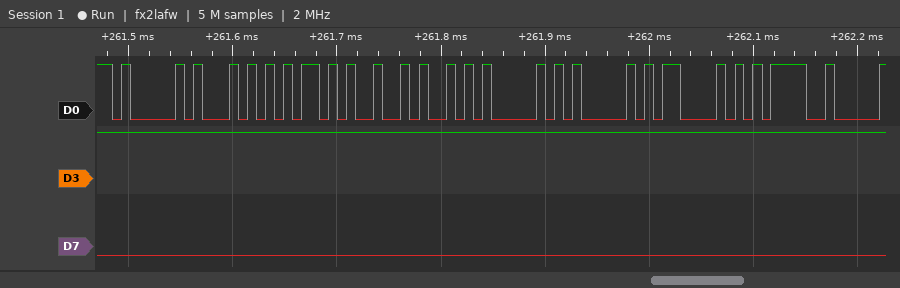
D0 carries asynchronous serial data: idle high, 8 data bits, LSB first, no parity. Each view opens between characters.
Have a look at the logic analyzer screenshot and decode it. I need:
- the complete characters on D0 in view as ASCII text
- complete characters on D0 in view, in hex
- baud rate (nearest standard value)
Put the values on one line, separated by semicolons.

"AT+JAAC="; 41, 54, 2B, 4A, 41, 41, 43, 3D; 115200 baud
